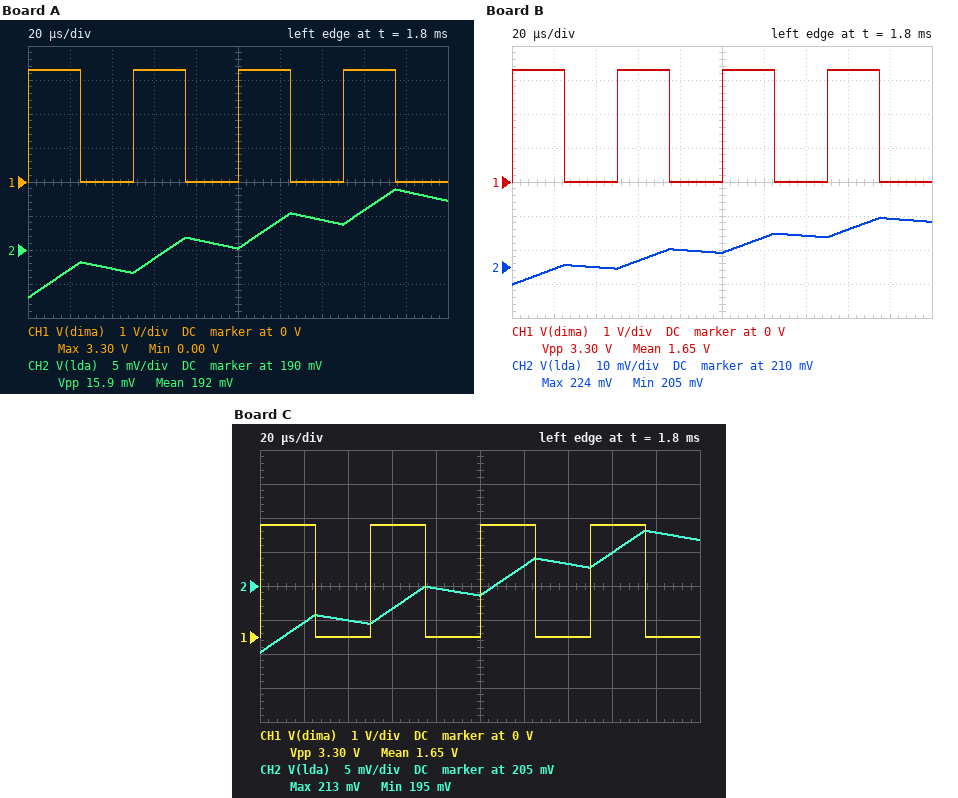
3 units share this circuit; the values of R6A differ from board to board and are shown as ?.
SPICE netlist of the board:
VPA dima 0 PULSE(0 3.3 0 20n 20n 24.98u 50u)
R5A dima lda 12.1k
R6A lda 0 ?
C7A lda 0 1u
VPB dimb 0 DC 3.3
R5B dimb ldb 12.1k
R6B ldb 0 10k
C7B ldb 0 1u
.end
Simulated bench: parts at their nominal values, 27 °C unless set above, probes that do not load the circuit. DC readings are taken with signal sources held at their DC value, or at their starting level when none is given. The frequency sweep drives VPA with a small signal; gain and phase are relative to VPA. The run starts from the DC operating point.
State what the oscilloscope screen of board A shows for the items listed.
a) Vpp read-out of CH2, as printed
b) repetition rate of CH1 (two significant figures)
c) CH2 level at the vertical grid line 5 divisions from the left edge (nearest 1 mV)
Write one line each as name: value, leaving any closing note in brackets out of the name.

Vpp read-out of CH2, as printed: 15.9 mV
repetition rate of CH1: 20 kHz
CH2 level at the vertical grid line 5 divisions from the left edge: 190 mV
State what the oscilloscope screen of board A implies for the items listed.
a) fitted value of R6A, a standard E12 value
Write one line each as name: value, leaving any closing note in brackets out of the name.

fitted value of R6A, a standard E12 value: 3.9 kΩ
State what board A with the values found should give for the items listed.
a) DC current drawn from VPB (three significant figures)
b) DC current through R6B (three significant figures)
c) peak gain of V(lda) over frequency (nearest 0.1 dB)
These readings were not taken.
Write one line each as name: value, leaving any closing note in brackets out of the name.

DC current drawn from VPB: 149 µA
DC current through R6B: 149 µA
peak gain of V(lda) over frequency: -12.3 dB
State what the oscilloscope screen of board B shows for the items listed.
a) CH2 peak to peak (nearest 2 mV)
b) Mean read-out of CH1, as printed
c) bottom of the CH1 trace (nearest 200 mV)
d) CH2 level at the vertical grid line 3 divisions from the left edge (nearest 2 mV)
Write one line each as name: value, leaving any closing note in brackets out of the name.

CH2 peak to peak: 20 mV
Mean read-out of CH1, as printed: 1.65 V
bottom of the CH1 trace: 0 V
CH2 level at the vertical grid line 3 divisions from the left edge: 212 mV
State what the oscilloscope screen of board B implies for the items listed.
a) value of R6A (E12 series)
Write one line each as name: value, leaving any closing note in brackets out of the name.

value of R6A: 8.2 kΩ
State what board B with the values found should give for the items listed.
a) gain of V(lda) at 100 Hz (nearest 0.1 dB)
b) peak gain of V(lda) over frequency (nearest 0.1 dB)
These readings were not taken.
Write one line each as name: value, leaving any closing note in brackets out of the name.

gain of V(lda) at 100 Hz: -18.1 dB
peak gain of V(lda) over frequency: -7.9 dB
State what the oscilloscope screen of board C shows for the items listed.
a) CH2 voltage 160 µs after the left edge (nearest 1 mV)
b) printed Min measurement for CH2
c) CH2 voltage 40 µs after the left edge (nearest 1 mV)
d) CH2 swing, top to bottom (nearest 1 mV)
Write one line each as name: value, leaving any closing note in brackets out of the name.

CH2 voltage 160 µs after the left edge: 210 mV
printed Min measurement for CH2: 195 mV
CH2 voltage 40 µs after the left edge: 200 mV
CH2 swing, top to bottom: 18 mV
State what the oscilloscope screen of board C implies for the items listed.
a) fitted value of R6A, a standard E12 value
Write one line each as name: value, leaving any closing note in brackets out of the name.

fitted value of R6A, a standard E12 value: 5.6 kΩ
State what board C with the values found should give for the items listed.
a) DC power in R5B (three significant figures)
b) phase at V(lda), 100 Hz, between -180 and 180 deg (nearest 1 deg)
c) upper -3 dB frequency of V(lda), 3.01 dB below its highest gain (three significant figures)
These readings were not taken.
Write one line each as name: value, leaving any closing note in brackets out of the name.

DC power in R5B: 270 µW
phase at V(lda), 100 Hz, between -180 and 180 deg: -67 deg
upper -3 dB frequency of V(lda), 3.01 dB below its highest gain: 41.6 Hz
